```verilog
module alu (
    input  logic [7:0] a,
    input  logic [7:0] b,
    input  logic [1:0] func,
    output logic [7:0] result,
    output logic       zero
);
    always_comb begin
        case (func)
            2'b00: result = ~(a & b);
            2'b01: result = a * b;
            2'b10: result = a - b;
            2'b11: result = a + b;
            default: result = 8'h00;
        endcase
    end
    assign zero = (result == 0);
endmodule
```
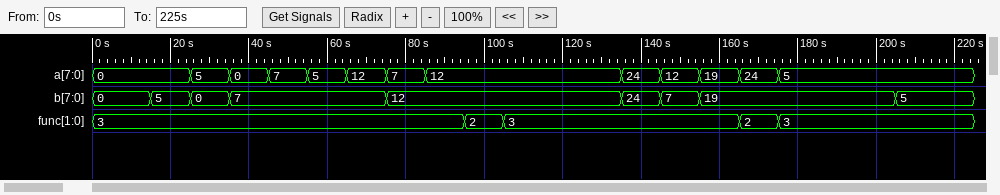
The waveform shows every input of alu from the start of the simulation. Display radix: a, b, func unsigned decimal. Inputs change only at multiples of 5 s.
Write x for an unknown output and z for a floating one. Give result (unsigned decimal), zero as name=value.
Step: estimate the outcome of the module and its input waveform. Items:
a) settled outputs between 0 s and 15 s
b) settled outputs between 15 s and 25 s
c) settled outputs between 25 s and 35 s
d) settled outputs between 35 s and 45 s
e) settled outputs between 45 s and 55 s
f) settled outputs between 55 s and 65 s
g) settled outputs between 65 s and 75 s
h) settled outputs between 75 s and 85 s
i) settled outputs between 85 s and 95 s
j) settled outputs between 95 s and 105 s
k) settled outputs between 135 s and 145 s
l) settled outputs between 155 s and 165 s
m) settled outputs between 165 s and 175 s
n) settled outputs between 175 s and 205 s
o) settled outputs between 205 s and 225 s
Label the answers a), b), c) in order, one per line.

a) result=0, zero=1
b) result=5, zero=0
c) result=5, zero=0
d) result=7, zero=0
e) result=14, zero=0
f) result=12, zero=0
g) result=19, zero=0
h) result=19, zero=0
i) result=24, zero=0
j) result=0, zero=1
k) result=48, zero=0
l) result=38, zero=0
m) result=5, zero=0
n) result=24, zero=0
o) result=10, zero=0
